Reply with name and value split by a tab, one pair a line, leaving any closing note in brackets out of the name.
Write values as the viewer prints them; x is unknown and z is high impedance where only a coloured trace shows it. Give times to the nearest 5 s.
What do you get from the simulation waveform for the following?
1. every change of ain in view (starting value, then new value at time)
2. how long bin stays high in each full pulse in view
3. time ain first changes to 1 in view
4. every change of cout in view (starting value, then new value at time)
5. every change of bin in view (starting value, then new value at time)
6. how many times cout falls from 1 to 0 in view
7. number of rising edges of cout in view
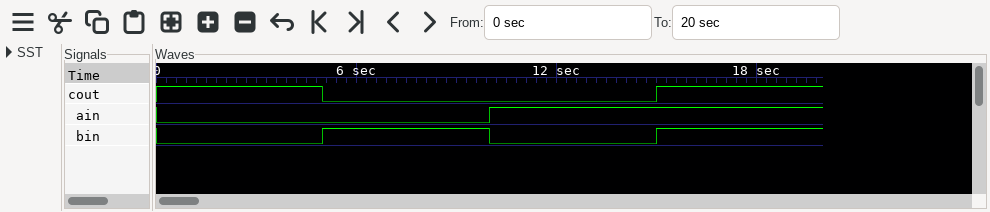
every change of ain in view	0, 1 at 10 s
how long bin stays high in each full pulse in view	5 s
time ain first changes to 1 in view	10 s
every change of cout in view	1, 0 at 5 s, 1 at 15 s
every change of bin in view	0, 1 at 5 s, 0 at 10 s, 1 at 15 s
how many times cout falls from 1 to 0 in view	1
number of rising edges of cout in view	1
